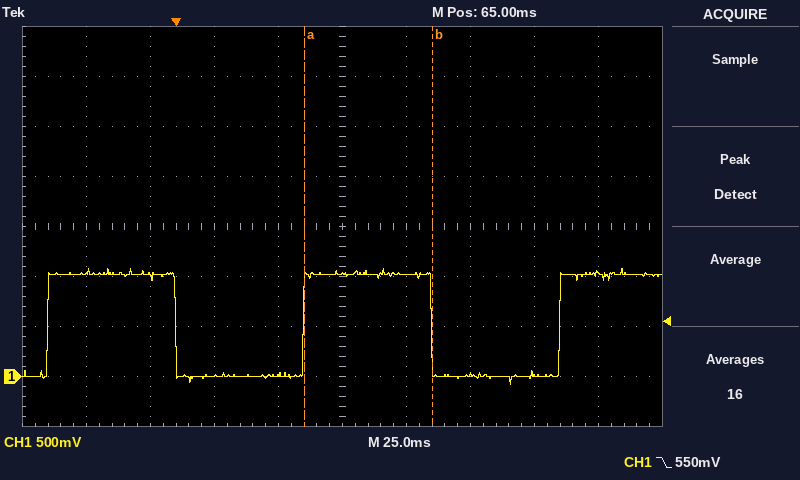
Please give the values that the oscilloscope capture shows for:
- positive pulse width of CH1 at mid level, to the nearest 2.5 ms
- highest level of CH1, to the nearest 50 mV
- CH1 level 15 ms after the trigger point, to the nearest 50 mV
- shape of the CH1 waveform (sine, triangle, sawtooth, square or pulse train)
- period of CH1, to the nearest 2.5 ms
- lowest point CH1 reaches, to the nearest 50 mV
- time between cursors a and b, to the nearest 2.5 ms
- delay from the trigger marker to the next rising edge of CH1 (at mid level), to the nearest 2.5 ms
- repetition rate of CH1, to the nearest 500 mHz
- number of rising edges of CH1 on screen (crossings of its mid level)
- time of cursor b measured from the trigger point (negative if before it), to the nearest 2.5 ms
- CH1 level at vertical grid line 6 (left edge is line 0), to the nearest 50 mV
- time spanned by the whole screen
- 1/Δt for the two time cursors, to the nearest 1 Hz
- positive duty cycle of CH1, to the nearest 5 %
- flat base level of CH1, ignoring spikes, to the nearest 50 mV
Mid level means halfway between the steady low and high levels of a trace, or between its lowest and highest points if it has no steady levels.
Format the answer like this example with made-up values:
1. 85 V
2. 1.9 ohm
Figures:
1. 50.0 ms
2. 1.10 V
3. 0 mV
4. square
5. 100.0 ms
6. -100 mV
7. 50.0 ms
8. 50.0 ms
9. 10.0 Hz
10. 3
11. +100.0 ms
12. 1.00 V
13. 250 ms
14. 20 Hz
15. 50 %
16. 0 mV
